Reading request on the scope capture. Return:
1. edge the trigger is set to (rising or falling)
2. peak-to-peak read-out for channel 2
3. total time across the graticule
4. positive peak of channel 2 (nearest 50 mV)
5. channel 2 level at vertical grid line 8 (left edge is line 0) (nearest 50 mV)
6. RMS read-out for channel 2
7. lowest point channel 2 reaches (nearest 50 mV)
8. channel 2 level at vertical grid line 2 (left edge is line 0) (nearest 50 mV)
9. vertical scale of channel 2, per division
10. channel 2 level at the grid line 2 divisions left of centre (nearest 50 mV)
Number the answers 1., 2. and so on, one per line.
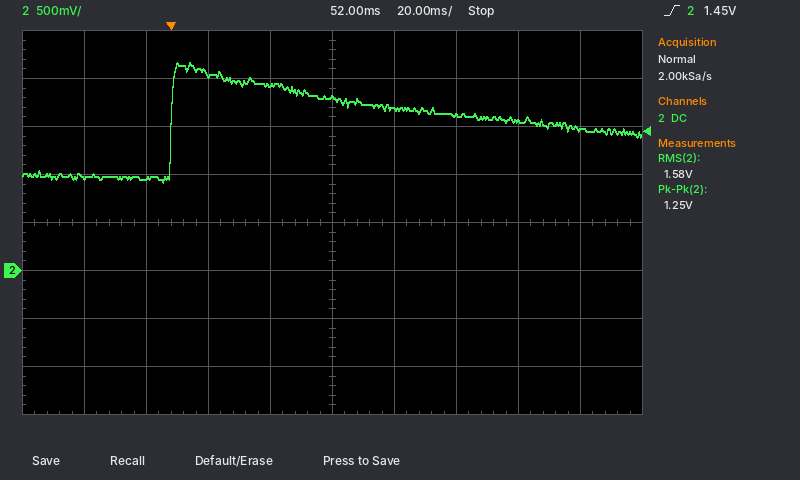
1. rising
2. 1.25 V
3. 200 ms
4. 2.15 V
5. 1.55 V
6. 1.58 V
7. 900 mV
8. 950 mV
9. 500 mV
10. 2.05 V
